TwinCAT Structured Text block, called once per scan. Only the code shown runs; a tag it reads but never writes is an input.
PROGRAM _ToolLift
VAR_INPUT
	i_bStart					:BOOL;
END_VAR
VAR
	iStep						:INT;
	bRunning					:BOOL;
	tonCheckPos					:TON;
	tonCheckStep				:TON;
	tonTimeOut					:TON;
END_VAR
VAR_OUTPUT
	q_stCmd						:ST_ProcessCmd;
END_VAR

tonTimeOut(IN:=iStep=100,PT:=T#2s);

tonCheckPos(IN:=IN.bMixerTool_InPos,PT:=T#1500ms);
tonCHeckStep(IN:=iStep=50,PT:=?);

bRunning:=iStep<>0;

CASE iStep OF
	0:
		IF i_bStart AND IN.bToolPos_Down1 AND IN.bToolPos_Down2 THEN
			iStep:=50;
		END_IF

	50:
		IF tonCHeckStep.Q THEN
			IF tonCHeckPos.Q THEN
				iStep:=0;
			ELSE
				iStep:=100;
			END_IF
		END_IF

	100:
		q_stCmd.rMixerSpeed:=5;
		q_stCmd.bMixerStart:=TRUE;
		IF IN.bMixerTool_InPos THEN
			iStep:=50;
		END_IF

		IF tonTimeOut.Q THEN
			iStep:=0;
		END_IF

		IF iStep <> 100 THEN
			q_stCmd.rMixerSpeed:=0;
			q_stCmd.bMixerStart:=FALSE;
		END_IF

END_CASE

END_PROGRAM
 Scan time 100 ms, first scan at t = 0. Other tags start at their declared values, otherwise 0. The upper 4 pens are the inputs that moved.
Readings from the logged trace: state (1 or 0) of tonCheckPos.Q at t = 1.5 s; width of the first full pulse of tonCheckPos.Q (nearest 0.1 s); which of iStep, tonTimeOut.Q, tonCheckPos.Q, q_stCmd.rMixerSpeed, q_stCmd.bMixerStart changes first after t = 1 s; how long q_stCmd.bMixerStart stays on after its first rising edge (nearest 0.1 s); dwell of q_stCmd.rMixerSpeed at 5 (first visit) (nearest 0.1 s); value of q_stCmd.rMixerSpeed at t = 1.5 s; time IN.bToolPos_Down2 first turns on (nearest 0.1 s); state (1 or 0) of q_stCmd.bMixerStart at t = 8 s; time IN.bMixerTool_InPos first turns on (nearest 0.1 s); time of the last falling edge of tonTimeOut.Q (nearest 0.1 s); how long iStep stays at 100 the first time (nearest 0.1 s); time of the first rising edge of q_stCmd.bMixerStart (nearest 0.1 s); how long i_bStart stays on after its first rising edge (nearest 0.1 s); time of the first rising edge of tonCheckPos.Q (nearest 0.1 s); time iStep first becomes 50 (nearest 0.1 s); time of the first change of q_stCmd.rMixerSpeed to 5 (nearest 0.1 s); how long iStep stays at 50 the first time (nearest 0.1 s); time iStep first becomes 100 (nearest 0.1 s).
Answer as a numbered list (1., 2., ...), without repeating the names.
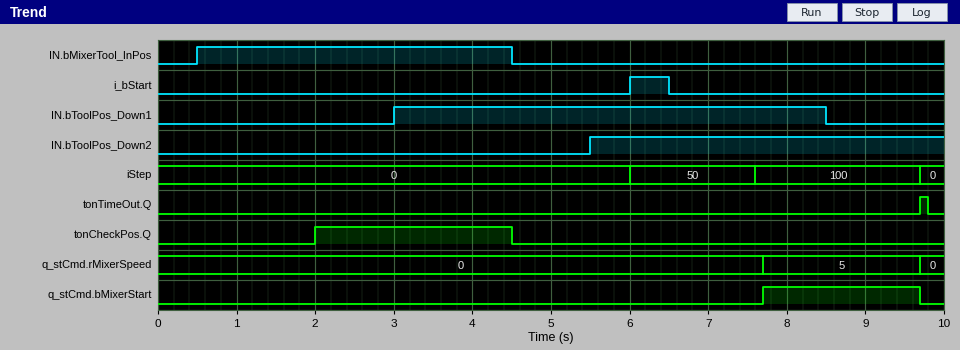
1. 0
2. 2.5 s
3. tonCheckPos.Q
4. 2.0 s
5. 2.0 s
6. 0
7. 5.5 s
8. 1
9. 0.5 s
10. 9.8 s
11. 2.1 s
12. 7.7 s
13. 0.5 s
14. 2.0 s
15. 6.0 s
16. 7.7 s
17. 1.6 s
18. 7.6 s
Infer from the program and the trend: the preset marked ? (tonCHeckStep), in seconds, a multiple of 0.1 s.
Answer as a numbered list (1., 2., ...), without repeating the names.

1. 1.5 s
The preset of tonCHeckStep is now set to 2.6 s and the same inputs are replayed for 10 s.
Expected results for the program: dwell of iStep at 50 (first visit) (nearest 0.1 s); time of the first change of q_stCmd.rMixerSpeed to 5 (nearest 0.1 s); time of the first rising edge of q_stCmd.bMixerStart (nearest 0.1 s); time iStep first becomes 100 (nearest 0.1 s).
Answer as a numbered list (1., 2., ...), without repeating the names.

1. 2.7 s
2. 8.8 s
3. 8.8 s
4. 8.7 s
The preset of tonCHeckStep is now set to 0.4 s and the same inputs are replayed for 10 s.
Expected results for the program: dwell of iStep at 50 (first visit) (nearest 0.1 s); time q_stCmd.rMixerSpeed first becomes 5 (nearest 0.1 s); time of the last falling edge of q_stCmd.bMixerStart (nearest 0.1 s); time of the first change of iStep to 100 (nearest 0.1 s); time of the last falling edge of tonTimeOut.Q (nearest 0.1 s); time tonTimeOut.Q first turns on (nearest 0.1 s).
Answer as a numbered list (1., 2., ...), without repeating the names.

1. 0.5 s
2. 6.6 s
3. 8.6 s
4. 6.5 s
5. 8.7 s
6. 8.6 s
